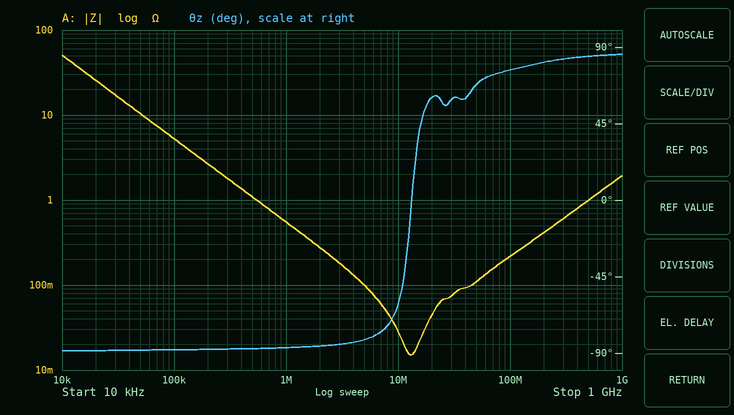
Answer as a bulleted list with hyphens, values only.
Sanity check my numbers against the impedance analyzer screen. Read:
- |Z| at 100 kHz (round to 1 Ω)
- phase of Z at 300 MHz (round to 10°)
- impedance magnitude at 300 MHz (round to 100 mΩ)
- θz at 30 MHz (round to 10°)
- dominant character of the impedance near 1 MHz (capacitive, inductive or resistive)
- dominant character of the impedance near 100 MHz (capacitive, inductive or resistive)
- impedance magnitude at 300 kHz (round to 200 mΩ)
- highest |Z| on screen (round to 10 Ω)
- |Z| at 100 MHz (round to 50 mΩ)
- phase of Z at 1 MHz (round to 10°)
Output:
- 5 Ω
- 80°
- 600 mΩ
- 60°
- capacitive
- inductive
- 1.8 Ω
- 50 Ω
- 200 mΩ
- -90°
